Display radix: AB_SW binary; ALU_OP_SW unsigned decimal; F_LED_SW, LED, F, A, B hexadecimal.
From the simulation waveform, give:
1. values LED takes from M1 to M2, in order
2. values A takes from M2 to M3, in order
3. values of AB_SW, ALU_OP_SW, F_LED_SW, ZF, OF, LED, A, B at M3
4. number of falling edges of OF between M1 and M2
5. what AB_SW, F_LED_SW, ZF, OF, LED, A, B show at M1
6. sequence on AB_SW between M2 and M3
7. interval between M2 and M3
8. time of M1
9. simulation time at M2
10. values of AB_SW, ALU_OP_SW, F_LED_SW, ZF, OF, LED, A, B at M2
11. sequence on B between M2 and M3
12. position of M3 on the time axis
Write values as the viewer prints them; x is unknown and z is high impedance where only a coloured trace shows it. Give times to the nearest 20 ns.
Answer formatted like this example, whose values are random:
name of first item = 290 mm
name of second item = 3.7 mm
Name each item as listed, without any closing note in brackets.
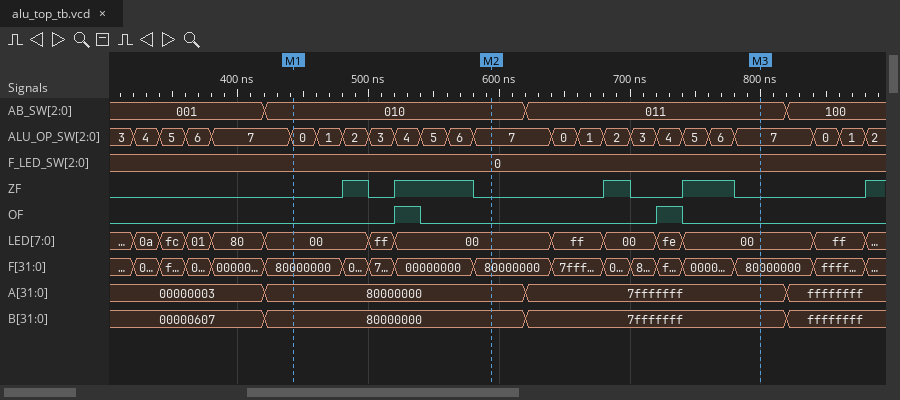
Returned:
values LED takes from M1 to M2, in order = 00, ff, 00
values A takes from M2 to M3, in order = 80000000, 7fffffff
values of AB_SW, ALU_OP_SW, F_LED_SW, ZF, OF, LED, A, B at M3 = AB_SW=011, ALU_OP_SW=7, F_LED_SW=0, ZF=0, OF=0, LED=00, A=7fffffff, B=7fffffff
number of falling edges of OF between M1 and M2 = 1
what AB_SW, F_LED_SW, ZF, OF, LED, A, B show at M1 = AB_SW=010, F_LED_SW=0, ZF=0, OF=0, LED=00, A=80000000, B=80000000
sequence on AB_SW between M2 and M3 = 010, 011
interval between M2 and M3 = 200 ns
time of M1 = 440 ns
simulation time at M2 = 600 ns
values of AB_SW, ALU_OP_SW, F_LED_SW, ZF, OF, LED, A, B at M2 = AB_SW=010, ALU_OP_SW=7, F_LED_SW=0, ZF=0, OF=0, LED=00, A=80000000, B=80000000
sequence on B between M2 and M3 = 80000000, 7fffffff
position of M3 on the time axis = 800 ns
